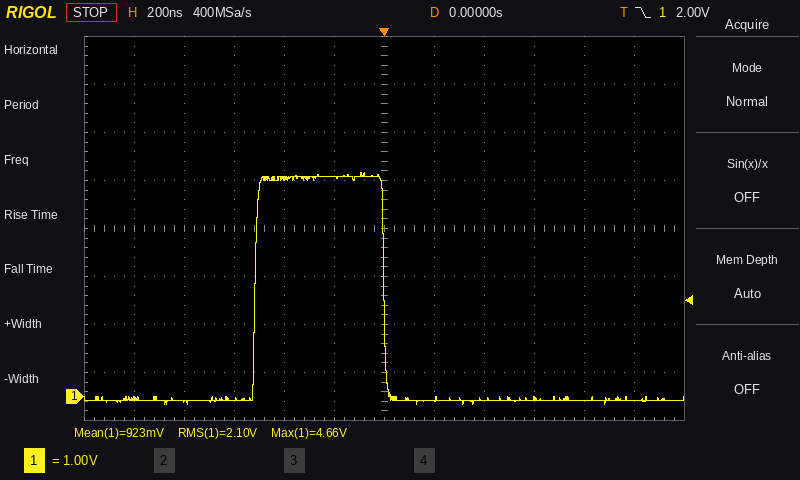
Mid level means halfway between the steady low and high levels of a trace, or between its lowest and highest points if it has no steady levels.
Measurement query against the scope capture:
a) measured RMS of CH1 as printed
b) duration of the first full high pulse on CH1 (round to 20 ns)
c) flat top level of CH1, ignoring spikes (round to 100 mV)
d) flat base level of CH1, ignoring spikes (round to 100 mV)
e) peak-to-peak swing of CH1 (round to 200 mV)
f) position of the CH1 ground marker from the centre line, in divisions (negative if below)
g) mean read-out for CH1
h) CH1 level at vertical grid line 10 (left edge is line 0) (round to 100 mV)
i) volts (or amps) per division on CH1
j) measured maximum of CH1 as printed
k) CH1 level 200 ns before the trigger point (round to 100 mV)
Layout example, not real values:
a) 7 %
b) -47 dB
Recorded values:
a) 2.10 V
b) 520 ns
c) 4.6 V
d) -100 mV
e) 4.8 V
f) -3.5 div
g) 923 mV
h) -100 mV
i) 1 V
j) 4.66 V
k) 4.6 V
